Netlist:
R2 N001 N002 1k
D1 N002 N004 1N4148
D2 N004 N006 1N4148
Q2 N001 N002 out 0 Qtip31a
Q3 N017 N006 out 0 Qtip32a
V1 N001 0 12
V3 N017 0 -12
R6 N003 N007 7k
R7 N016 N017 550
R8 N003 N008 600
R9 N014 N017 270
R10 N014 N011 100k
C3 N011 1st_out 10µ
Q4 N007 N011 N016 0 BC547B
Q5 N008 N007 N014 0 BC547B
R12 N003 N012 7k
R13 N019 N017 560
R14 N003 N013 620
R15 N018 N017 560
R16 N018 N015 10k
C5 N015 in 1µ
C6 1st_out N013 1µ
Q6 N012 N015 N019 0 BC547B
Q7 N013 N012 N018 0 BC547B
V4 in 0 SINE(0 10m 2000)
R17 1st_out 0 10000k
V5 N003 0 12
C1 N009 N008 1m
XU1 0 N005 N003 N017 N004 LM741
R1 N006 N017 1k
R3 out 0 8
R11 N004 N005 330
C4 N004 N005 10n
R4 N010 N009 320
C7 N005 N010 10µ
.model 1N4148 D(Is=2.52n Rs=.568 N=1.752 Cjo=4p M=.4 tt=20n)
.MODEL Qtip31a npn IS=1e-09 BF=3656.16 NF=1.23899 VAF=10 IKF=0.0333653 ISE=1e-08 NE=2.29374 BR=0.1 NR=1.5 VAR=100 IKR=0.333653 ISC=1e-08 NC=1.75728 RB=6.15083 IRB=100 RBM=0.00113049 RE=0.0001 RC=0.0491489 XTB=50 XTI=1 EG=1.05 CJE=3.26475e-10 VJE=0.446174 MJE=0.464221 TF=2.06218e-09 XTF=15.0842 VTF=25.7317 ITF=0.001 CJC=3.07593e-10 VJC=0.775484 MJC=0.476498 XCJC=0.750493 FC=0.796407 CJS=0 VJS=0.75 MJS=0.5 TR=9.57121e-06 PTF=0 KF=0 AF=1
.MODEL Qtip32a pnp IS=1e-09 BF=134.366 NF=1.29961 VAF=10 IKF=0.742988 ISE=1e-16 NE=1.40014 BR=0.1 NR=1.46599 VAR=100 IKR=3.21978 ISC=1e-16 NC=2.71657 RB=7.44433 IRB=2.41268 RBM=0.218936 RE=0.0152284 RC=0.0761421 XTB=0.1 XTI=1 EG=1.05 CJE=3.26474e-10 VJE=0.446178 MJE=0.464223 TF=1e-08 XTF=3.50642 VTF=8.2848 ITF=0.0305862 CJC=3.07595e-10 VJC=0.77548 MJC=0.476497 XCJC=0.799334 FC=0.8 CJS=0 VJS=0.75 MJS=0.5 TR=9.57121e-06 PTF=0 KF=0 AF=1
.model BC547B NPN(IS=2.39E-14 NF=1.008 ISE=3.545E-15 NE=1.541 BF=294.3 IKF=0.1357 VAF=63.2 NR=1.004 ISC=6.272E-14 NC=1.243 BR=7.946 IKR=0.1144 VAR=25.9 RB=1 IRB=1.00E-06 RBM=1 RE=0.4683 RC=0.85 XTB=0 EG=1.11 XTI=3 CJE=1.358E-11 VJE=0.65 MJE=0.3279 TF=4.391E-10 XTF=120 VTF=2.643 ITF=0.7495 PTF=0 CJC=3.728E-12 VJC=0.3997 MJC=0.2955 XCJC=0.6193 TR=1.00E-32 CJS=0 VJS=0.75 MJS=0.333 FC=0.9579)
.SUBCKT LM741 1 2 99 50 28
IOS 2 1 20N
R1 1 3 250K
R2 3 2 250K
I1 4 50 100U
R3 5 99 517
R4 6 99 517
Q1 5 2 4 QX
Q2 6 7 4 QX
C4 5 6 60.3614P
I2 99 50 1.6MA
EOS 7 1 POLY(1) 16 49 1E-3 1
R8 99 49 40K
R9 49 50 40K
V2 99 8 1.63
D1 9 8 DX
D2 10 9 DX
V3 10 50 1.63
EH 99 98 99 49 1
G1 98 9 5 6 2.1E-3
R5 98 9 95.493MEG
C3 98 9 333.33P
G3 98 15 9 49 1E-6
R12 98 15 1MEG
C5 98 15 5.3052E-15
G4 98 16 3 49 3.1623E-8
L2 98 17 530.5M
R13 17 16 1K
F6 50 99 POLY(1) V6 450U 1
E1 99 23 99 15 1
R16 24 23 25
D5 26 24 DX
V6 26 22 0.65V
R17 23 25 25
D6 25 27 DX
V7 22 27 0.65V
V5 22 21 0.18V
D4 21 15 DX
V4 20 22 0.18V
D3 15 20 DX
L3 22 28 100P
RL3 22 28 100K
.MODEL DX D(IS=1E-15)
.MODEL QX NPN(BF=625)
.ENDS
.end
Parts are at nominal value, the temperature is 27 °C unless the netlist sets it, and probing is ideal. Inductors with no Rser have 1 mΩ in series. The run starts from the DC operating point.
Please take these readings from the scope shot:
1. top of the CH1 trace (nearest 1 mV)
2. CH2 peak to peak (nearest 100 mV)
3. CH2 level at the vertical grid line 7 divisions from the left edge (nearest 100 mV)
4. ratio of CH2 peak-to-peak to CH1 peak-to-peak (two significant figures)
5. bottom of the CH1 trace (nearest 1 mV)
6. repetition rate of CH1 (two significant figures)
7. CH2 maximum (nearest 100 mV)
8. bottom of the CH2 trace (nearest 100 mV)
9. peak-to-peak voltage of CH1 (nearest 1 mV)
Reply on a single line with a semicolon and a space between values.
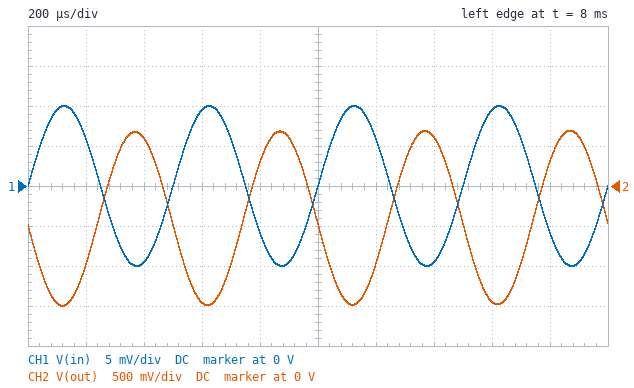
10 mV; 2.2 V; 600 mV; 110; -10 mV; 2.0 kHz; 700 mV; -1.5 V; 20 mV
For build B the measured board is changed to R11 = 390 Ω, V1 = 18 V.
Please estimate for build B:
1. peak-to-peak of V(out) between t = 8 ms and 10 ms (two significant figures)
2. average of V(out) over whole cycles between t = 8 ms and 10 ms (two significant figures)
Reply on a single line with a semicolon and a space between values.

2.6 V; -450 mV
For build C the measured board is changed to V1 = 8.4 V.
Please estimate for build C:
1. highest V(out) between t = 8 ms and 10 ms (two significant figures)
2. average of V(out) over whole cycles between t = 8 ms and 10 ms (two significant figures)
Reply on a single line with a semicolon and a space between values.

670 mV; -420 mV
